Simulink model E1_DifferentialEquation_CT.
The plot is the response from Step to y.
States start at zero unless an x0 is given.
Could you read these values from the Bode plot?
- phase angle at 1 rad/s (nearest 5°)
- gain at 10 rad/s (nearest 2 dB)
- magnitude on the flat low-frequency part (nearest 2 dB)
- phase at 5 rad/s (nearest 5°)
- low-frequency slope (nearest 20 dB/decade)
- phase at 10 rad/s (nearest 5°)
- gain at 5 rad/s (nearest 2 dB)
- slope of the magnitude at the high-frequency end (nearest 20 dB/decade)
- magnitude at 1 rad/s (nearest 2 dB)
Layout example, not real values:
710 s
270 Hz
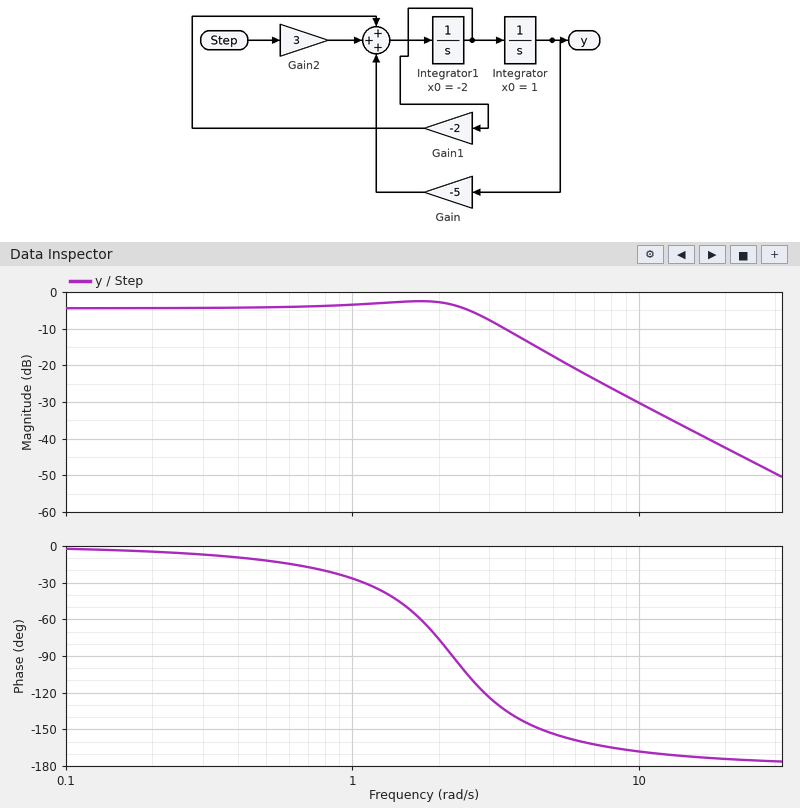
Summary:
-25°
-30 dB
-4 dB
-155°
0 dB/decade
-170°
-18 dB
-40 dB/decade
-4 dB
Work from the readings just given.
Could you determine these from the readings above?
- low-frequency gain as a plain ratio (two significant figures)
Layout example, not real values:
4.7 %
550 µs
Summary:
0.63
